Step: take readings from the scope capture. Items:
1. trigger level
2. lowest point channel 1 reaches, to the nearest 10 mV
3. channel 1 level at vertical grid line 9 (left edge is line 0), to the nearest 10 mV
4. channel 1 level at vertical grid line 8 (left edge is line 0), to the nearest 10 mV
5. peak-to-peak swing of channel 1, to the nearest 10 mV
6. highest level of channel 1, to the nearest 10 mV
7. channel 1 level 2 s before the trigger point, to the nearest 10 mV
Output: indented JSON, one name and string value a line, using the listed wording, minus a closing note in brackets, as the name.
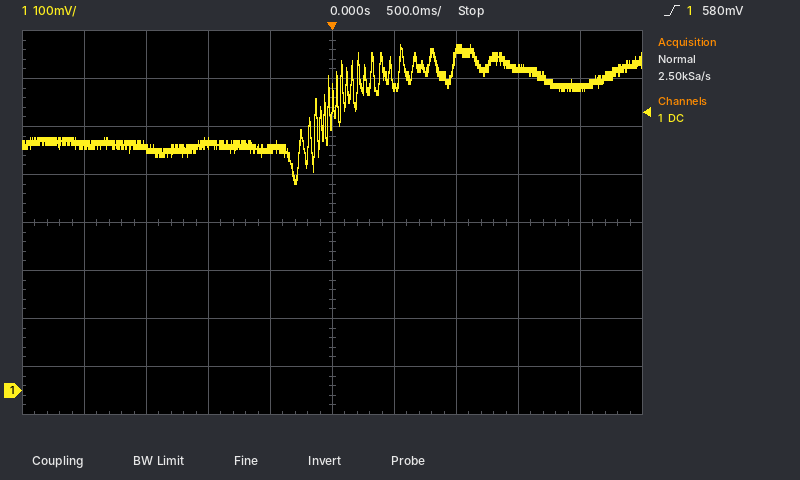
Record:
{
  "trigger level": "580 mV",
  "lowest point channel 1 reaches, to the nearest 10 mV": "430 mV",
  "channel 1 level at vertical grid line 9 (left edge is line 0), to the nearest 10 mV": "630 mV",
  "channel 1 level at vertical grid line 8 (left edge is line 0), to the nearest 10 mV": "670 mV",
  "peak-to-peak swing of channel 1, to the nearest 10 mV": "290 mV",
  "highest level of channel 1, to the nearest 10 mV": "720 mV",
  "channel 1 level 2 s before the trigger point, to the nearest 10 mV": "510 mV"
}
